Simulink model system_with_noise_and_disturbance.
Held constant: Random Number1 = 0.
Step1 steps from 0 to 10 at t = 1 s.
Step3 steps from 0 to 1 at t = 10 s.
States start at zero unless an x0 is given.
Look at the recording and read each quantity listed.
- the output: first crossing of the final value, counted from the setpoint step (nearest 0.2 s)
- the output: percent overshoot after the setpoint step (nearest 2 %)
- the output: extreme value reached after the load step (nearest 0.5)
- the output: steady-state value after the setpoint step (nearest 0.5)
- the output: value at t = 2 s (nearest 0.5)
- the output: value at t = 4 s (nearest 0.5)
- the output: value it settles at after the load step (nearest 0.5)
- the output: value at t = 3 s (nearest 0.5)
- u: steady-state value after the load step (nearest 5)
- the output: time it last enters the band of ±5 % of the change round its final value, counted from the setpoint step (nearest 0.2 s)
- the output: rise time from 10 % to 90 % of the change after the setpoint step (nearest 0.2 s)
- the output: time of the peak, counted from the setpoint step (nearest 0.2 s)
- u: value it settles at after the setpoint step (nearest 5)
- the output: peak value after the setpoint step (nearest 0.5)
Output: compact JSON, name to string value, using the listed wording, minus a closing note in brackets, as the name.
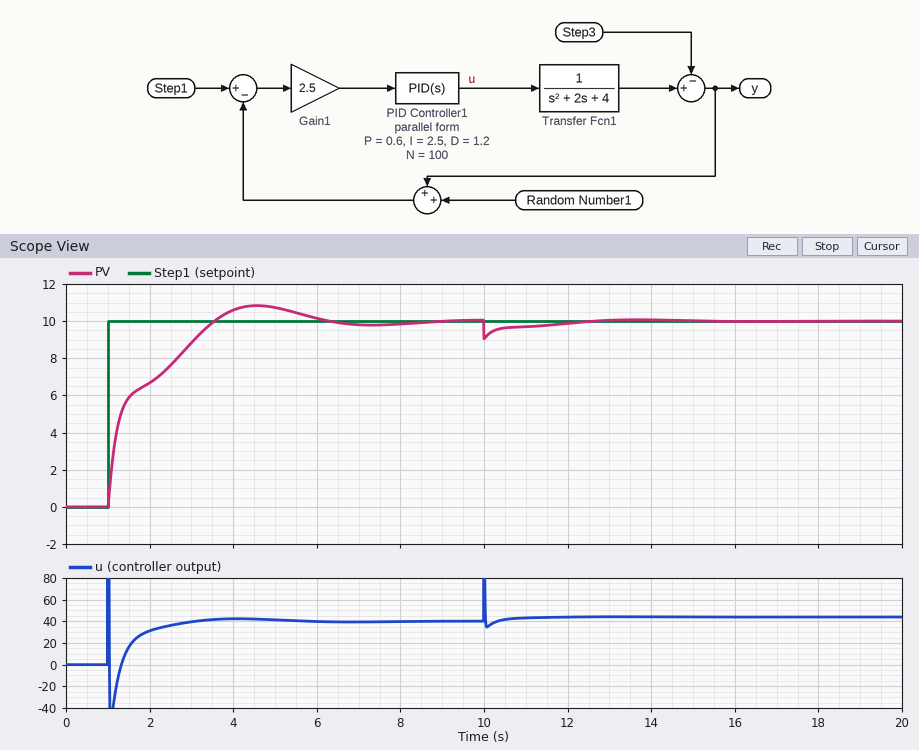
{"the output: first crossing of the final value, counted from the setpoint step": "2.6 s", "the output: percent overshoot after the setpoint step": "8 %", "the output: extreme value reached after the load step": "9.0", "the output: steady-state value after the setpoint step": "10.0", "the output: value at t = 2 s": "6.5", "the output: value at t = 4 s": "10.5", "the output: value it settles at after the load step": "10.0", "the output: value at t = 3 s": "9.0", "u: steady-state value after the load step": "45", "the output: time it last enters the band of ±5 % of the change round its final value, counted from the setpoint step": "4.4 s", "the output: rise time from 10 % to 90 % of the change after the setpoint step": "2.0 s", "the output: time of the peak, counted from the setpoint step": "3.6 s", "u: value it settles at after the setpoint step": "40", "the output: peak value after the setpoint step": "11.0"}
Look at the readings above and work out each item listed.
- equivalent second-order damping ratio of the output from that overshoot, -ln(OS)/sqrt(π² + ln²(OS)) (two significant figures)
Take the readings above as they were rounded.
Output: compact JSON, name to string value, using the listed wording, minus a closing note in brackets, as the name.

{"equivalent second-order damping ratio of the output from that overshoot, -ln(OS)/sqrt(π² + ln²(OS))": "0.63"}
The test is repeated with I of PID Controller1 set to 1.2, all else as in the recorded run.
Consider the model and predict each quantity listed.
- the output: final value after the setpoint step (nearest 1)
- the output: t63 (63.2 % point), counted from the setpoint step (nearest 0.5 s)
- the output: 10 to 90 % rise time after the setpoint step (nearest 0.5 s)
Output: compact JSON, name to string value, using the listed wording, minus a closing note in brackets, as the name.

{"the output: final value after the setpoint step": "10", "the output: t63 (63.2 % point), counted from the setpoint step": "2.0 s", "the output: 10 to 90 % rise time after the setpoint step": "3.5 s"}
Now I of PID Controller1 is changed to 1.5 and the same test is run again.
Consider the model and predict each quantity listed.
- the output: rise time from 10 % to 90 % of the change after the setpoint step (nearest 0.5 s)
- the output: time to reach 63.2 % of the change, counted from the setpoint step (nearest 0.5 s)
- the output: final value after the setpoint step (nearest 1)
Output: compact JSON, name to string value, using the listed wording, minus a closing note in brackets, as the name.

{"the output: rise time from 10 % to 90 % of the change after the setpoint step": "3.0 s", "the output: time to reach 63.2 % of the change, counted from the setpoint step": "1.5 s", "the output: final value after the setpoint step": "10"}
